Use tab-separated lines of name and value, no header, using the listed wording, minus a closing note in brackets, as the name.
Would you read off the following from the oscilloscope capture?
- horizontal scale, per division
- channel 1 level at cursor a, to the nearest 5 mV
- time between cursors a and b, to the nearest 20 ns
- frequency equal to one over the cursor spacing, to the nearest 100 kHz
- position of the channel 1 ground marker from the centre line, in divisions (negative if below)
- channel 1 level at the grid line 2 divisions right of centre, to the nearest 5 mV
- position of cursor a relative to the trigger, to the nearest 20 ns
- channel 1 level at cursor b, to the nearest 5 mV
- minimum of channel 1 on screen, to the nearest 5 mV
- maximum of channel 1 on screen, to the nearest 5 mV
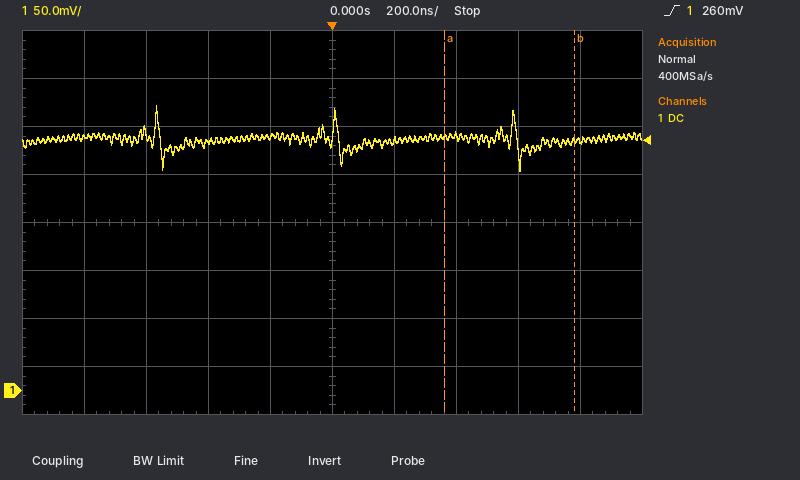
horizontal scale, per division	200 ns
channel 1 level at cursor a, to the nearest 5 mV	265 mV
time between cursors a and b, to the nearest 20 ns	420 ns
frequency equal to one over the cursor spacing, to the nearest 100 kHz	2.4 MHz
position of the channel 1 ground marker from the centre line, in divisions	-3.5 div
channel 1 level at the grid line 2 divisions right of centre, to the nearest 5 mV	265 mV
position of cursor a relative to the trigger, to the nearest 20 ns	+360 ns
channel 1 level at cursor b, to the nearest 5 mV	260 mV
minimum of channel 1 on screen, to the nearest 5 mV	230 mV
maximum of channel 1 on screen, to the nearest 5 mV	295 mV
